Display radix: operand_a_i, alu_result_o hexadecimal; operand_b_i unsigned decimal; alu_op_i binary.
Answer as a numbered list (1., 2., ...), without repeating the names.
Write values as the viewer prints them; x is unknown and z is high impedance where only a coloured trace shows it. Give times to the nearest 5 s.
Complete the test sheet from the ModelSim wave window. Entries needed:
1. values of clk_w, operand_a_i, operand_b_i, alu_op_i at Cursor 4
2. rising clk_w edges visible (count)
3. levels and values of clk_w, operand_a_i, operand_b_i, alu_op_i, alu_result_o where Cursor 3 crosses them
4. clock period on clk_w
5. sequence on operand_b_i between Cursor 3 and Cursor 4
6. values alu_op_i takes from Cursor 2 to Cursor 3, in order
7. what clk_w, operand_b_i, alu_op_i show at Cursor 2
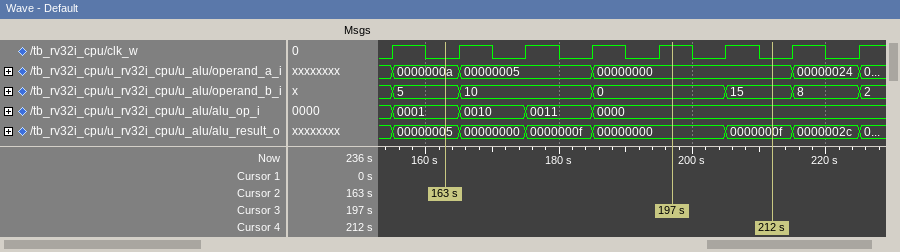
1. clk_w=0, operand_a_i=00000000, operand_b_i=15, alu_op_i=0000
2. 8
3. clk_w=1, operand_a_i=00000000, operand_b_i=0, alu_op_i=0000, alu_result_o=00000000
4. 10 s
5. 0, 15
6. 0001, 0010, 0011, 0000
7. clk_w=0, operand_b_i=5, alu_op_i=0001
